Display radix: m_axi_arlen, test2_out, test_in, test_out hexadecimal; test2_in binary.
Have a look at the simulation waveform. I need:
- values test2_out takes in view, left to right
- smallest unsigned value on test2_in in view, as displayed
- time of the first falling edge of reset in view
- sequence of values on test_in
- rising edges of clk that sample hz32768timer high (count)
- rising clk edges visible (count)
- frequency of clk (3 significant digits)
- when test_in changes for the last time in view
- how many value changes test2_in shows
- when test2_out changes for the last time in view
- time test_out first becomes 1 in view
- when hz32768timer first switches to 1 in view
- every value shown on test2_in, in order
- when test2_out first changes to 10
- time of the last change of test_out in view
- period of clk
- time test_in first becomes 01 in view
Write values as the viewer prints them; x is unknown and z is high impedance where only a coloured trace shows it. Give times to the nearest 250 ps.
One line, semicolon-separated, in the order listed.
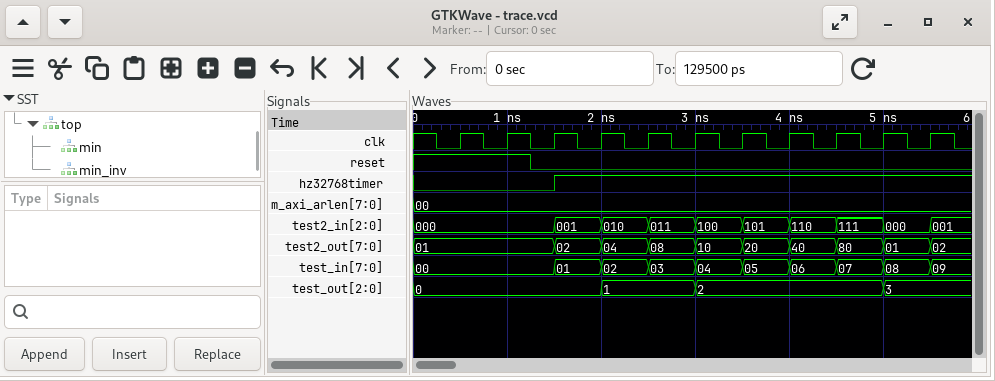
01, 02, 04, 08, 10, 20, 40, 80, 01, 02; 000; 1250 ps; 00, 01, 02, 03, 04, 05, 06, 07, 08, 09; 8; 11; 2.00 GHz; 5500 ps; 9; 5500 ps; 2000 ps; 1500 ps; 000, 001, 010, 011, 100, 101, 110, 111, 000, 001; 3000 ps; 5000 ps; 500 ps; 1500 ps
